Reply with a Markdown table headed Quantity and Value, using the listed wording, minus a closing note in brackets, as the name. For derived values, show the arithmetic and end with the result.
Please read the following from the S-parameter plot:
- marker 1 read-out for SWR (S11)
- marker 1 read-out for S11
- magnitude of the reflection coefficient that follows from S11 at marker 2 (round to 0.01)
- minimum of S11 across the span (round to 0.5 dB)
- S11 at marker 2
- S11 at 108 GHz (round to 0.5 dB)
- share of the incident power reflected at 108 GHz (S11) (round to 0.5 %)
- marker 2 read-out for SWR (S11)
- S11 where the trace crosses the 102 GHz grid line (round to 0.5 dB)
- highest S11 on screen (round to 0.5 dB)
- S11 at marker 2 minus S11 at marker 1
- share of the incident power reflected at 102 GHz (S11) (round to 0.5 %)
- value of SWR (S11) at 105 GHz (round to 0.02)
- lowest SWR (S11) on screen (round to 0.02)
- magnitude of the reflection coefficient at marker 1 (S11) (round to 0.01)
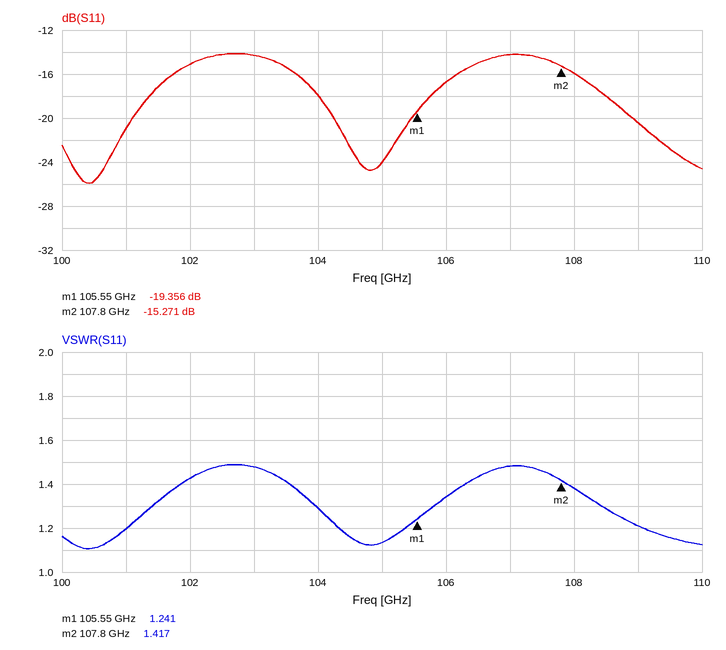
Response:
| Quantity | Value |
|---|---|
| marker 1 read-out for SWR | 1.241 |
| marker 1 read-out for S11 | -19.356 dB |
| magnitude of the reflection coefficient that follows from S11 at marker 2 | 10^(-15.271/20) ≈ 0.17 |
| minimum of S11 across the span | -26.0 dB |
| S11 at marker 2 | -15.271 dB |
| S11 at 108 GHz | -16.0 dB |
| share of the incident power reflected at 108 GHz (S11) | 10^(-16/10) ≈ 2.5 % |
| marker 2 read-out for SWR | 1.417 |
| S11 where the trace crosses the 102 GHz grid line | -15.0 dB |
| highest S11 on screen | -14.0 dB |
| S11 at marker 2 minus S11 at marker 1 | -15.271 − (-19.356) = 4.085 dB |
| share of the incident power reflected at 102 GHz (S11) | 10^(-15/10) ≈ 3.16 %, so 3.0 % to the nearest 0.5 % |
| value of SWR (S11) at 105 GHz | 1.14 |
| lowest SWR (S11) on screen | 1.10 |
| magnitude of the reflection coefficient at marker 1 (S11) | 10^(-19.356/20) ≈ 0.11 |
